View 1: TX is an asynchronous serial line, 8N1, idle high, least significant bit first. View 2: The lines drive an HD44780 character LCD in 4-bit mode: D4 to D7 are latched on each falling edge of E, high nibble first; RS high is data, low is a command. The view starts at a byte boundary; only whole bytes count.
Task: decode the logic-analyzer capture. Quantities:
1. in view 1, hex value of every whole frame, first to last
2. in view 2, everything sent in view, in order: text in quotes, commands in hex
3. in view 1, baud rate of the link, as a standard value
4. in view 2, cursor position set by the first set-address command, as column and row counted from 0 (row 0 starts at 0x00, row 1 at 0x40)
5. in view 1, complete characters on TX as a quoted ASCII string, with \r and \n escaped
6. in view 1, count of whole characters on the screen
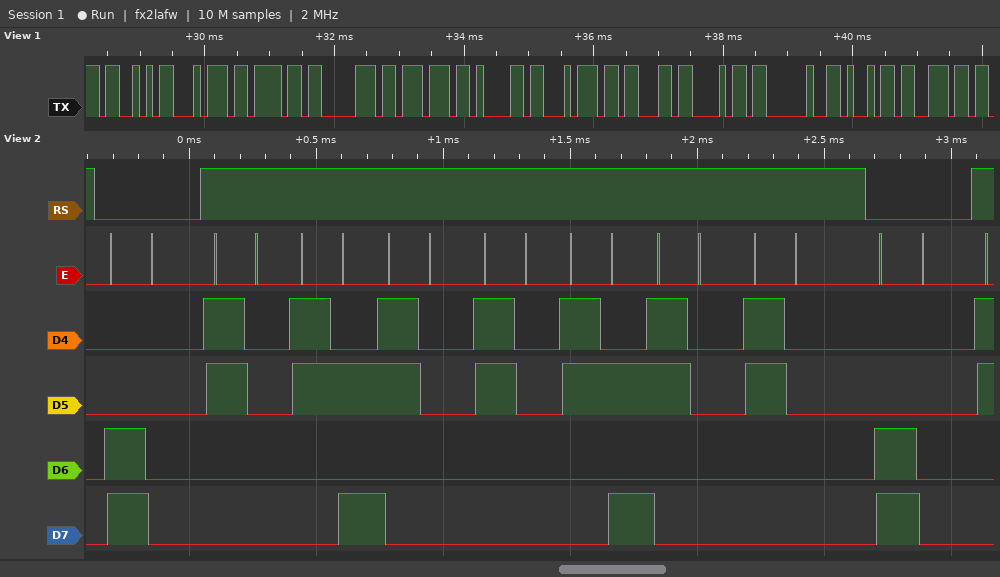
53 74 6F 70 77 61 74 63 68 20 69 6E
0xC0 "0:00:00" 0xC0
9600 baud
column 0, row 1
"Stopwatch in"
12
